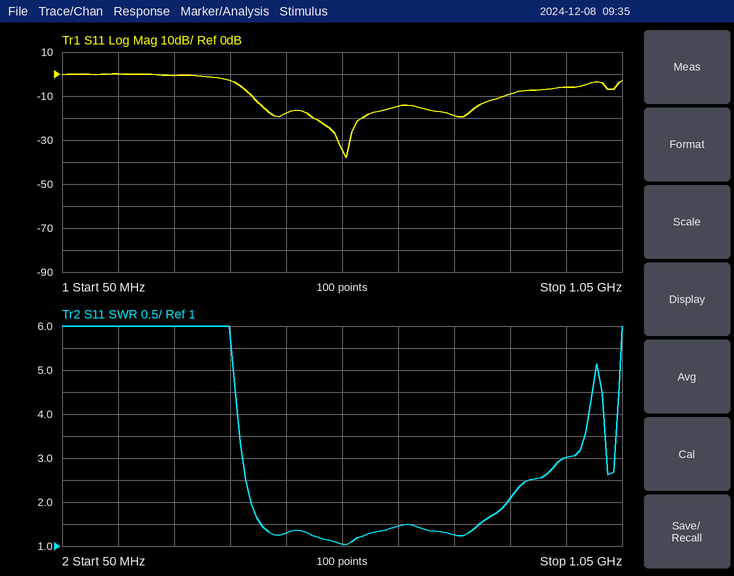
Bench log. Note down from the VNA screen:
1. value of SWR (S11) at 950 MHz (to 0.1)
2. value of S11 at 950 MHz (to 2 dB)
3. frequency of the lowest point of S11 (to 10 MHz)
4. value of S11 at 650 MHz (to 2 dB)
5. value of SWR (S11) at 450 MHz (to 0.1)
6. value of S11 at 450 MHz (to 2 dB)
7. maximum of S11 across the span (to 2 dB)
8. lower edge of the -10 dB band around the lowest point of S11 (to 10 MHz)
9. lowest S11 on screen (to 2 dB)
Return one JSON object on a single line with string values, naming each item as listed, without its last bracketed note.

{"value of SWR (S11) at 950 MHz": "3.0", "value of S11 at 950 MHz": "-6 dB", "frequency of the lowest point of S11": "560 MHz", "value of S11 at 650 MHz": "-14 dB", "value of SWR (S11) at 450 MHz": "1.3", "value of S11 at 450 MHz": "-18 dB", "maximum of S11 across the span": "0 dB", "lower edge of the -10 dB band around the lowest point of S11": "390 MHz", "lowest S11 on screen": "-38 dB"}
